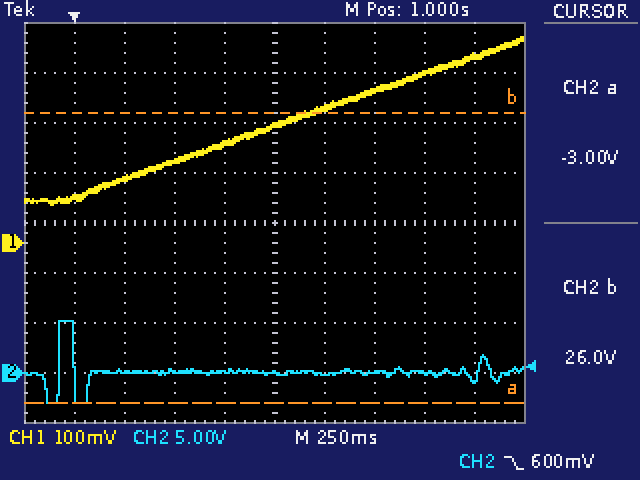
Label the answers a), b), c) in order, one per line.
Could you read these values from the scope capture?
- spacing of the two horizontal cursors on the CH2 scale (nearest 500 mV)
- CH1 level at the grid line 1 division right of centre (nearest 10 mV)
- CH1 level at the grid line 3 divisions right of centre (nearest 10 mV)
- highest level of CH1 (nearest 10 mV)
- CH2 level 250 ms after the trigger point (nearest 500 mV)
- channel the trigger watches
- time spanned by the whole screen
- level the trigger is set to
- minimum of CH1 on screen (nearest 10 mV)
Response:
a) 29.0 V
b) 270 mV
c) 340 mV
d) 410 mV
e) 0.0 V
f) CH2
g) 2.5 s
h) 600 mV
i) 80 mV
